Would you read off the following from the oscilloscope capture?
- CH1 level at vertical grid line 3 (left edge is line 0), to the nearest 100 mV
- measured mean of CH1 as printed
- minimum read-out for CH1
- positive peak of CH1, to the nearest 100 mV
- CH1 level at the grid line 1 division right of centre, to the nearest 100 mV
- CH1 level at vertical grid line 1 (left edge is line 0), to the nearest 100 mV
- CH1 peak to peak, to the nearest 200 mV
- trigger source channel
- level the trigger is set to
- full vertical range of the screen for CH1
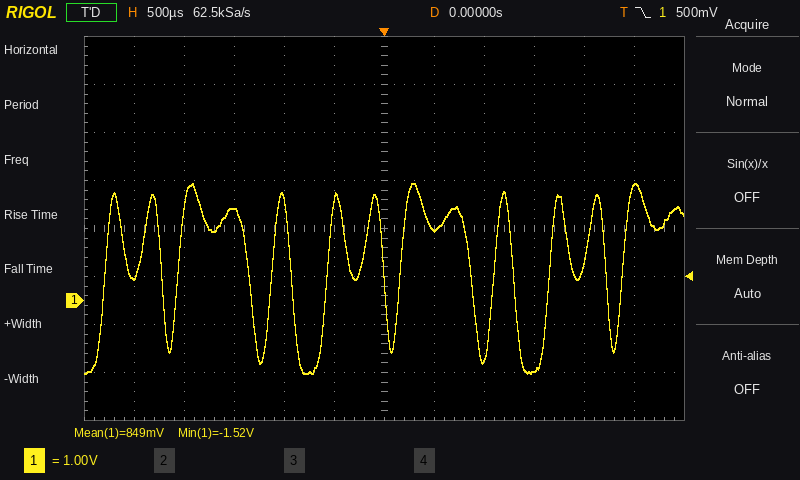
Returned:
1.9 V
849 mV
-1.52 V
2.4 V
1.5 V
500 mV
4.0 V
CH1
500 mV
8 V
